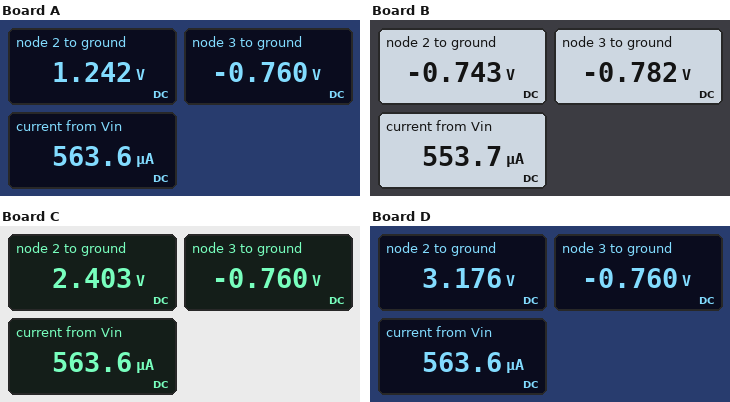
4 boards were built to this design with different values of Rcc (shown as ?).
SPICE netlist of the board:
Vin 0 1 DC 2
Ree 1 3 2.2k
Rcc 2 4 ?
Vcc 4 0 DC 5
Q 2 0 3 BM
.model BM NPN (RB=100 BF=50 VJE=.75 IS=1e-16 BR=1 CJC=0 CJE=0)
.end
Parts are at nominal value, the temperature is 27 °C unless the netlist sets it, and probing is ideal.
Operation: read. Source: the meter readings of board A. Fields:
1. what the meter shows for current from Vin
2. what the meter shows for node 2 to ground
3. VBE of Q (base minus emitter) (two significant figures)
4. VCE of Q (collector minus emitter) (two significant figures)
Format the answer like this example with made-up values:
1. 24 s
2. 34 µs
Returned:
1. 563.6 µA
2. 1.242 V
3. 760 mV
4. 2.0 V
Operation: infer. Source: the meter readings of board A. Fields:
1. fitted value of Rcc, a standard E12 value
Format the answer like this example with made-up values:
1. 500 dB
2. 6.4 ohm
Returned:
1. 6.8 kΩ
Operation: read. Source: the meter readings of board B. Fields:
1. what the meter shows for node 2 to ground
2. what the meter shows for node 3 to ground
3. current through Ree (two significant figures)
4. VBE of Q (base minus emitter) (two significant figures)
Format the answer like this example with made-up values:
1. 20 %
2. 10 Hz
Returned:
1. -0.743 V
2. -0.782 V
3. 550 µA
4. 780 mV
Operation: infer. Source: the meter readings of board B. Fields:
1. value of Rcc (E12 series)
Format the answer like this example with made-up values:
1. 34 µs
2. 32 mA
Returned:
1. 15 kΩ
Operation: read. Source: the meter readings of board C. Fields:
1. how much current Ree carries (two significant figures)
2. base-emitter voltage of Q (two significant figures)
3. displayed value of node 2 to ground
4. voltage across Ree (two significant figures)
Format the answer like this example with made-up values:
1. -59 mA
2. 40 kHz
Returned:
1. 560 µA
2. 760 mV
3. 2.403 V
4. 1.2 V
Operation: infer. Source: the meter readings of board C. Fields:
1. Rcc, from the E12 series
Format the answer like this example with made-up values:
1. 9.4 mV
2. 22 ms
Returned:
1. 4.7 kΩ
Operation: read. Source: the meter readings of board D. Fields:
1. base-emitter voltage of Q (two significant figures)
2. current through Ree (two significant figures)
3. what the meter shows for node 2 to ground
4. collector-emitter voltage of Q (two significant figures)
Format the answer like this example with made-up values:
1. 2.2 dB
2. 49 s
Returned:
1. 760 mV
2. 560 µA
3. 3.176 V
4. 3.9 V
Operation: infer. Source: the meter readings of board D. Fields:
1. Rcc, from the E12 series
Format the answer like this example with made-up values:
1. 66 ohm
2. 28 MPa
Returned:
1. 3.3 kΩ
